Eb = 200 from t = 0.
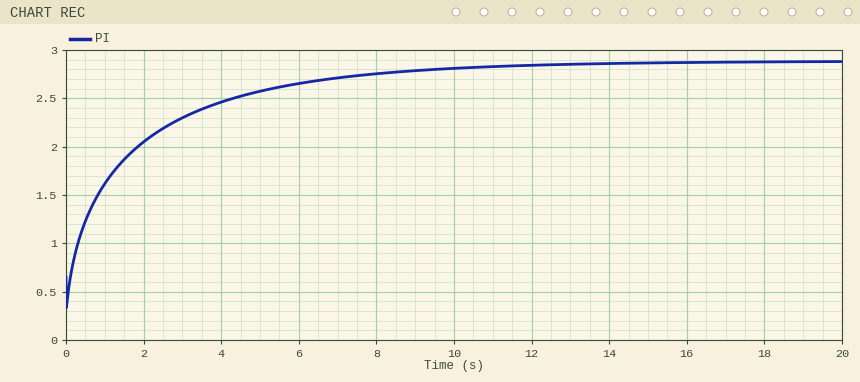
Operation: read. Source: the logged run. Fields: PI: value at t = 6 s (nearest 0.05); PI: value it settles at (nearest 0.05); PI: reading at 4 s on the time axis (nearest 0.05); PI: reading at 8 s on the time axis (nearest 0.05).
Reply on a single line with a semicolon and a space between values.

2.65; 2.90; 2.45; 2.75
